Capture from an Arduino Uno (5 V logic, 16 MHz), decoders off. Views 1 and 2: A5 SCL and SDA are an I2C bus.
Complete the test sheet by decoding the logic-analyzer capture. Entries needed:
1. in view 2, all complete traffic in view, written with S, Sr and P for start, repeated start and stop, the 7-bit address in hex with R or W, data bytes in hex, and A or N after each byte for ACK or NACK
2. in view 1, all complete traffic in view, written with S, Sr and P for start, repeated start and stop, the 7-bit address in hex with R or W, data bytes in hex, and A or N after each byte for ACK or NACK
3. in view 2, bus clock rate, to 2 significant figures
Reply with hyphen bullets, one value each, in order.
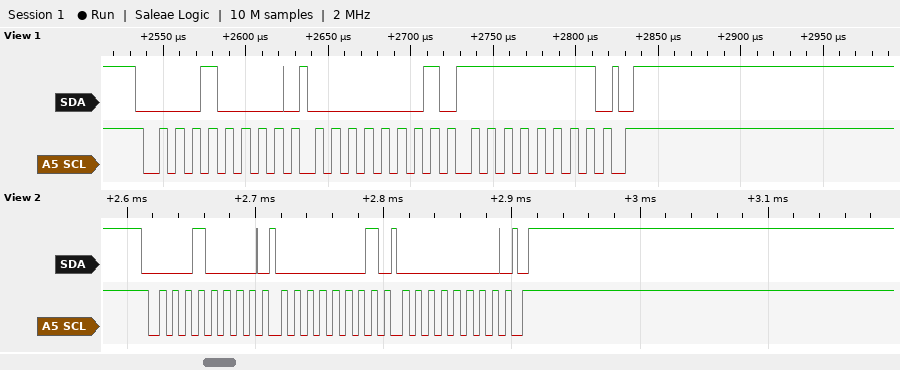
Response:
- S 08W A 01 A 00 A P
- S 08W A 01 A FF A P
- 100 kHz
